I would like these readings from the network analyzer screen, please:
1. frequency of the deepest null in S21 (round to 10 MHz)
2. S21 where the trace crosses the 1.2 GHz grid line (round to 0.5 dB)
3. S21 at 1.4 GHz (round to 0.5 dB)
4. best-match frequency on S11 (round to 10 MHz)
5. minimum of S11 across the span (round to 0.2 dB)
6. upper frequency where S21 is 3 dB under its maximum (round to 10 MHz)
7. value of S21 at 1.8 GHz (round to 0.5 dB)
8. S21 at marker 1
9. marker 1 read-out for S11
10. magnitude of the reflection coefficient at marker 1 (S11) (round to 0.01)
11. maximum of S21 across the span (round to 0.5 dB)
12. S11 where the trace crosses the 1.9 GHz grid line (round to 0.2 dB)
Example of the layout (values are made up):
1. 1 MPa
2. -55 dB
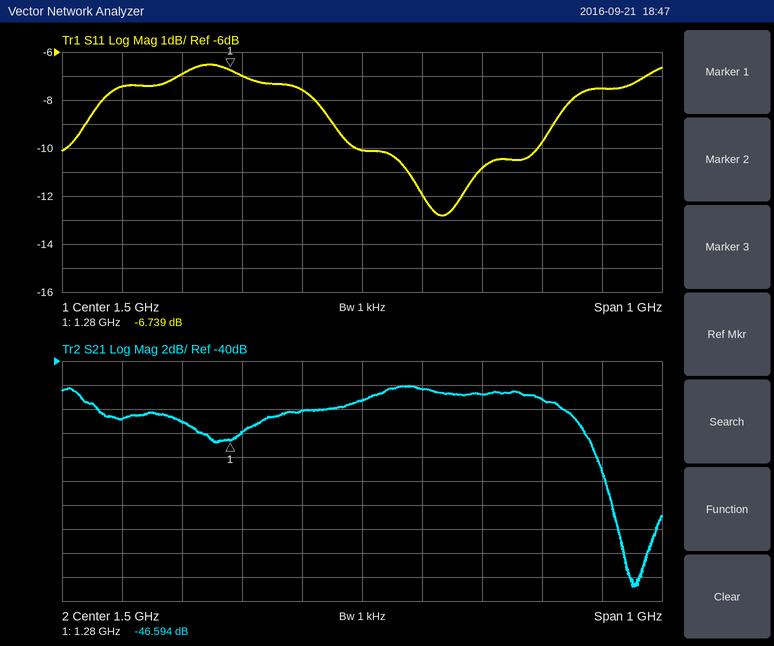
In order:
1. 1.95 GHz
2. -45.0 dB
3. -44.0 dB
4. 1.63 GHz
5. -12.8 dB
6. 1.86 GHz
7. -43.0 dB
8. -46.594 dB
9. -6.739 dB
10. 0.46
11. -42.0 dB
12. -7.6 dB
